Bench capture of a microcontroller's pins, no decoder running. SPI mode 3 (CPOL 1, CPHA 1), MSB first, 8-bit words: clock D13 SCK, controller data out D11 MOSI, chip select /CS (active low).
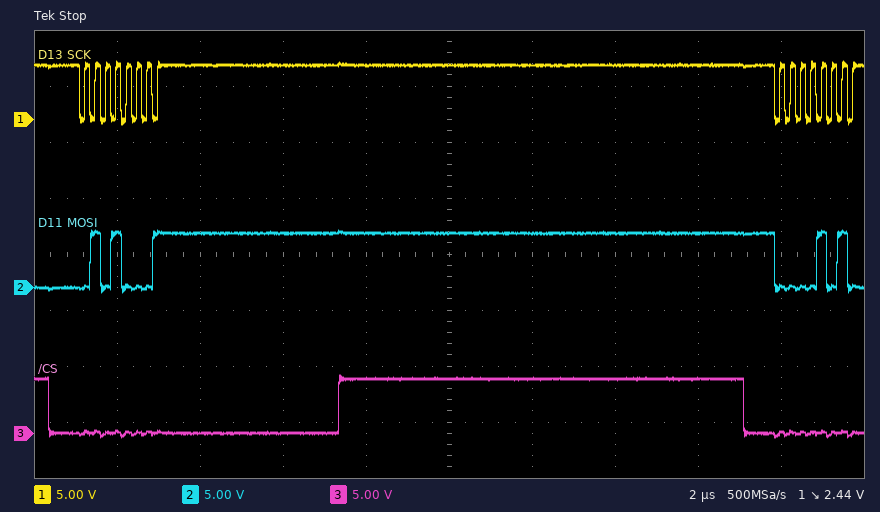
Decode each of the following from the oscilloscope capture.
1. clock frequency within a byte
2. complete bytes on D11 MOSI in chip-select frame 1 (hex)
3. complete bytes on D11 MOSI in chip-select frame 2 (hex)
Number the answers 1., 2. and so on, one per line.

1. 4 MHz
2. 51
3. 0A
